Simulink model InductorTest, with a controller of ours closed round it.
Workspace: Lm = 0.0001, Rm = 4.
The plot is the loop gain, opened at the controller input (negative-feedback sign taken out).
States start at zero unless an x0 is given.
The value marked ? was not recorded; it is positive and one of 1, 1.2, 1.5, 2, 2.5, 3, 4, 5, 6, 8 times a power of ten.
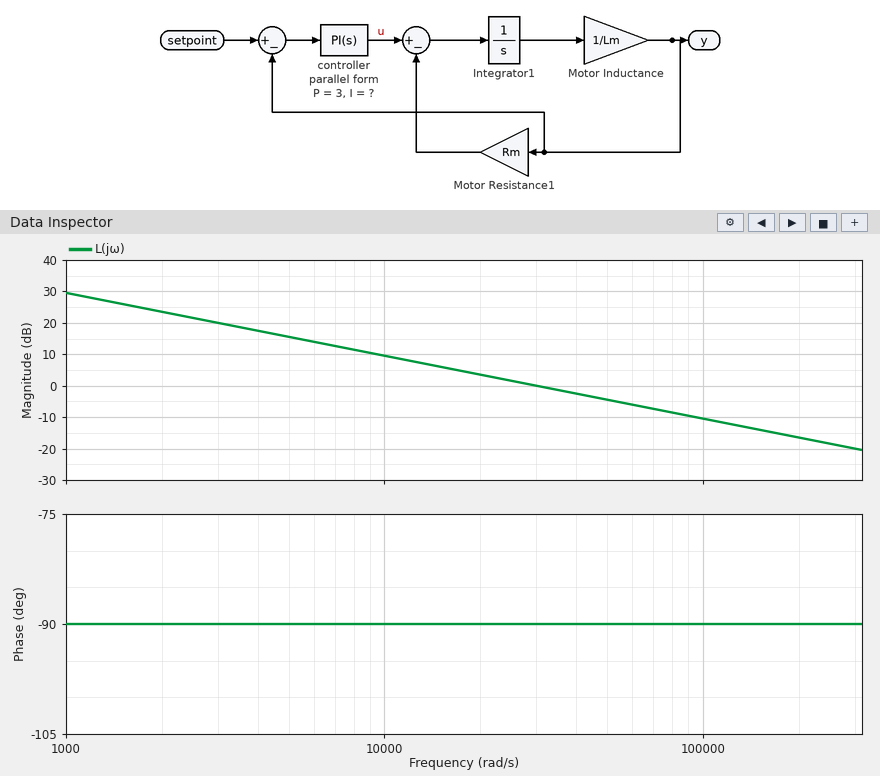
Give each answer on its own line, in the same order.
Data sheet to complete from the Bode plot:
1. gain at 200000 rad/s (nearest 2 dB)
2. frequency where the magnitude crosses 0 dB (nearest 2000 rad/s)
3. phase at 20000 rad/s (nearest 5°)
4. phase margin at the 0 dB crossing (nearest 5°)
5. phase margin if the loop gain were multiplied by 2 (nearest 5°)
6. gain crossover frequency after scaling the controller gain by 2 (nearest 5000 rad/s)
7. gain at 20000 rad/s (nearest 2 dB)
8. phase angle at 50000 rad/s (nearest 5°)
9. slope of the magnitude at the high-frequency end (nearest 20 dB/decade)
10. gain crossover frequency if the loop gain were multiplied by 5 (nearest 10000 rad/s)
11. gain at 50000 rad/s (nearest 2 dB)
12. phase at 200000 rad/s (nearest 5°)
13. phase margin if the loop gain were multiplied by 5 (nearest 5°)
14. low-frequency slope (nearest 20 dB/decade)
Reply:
-16 dB
30000 rad/s
-90°
90°
90°
60000 rad/s
4 dB
-90°
-20 dB/decade
150000 rad/s
-4 dB
-90°
90°
-20 dB/decade
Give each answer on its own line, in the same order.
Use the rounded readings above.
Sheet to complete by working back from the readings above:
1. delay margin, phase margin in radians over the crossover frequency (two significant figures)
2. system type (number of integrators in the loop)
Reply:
0.000052 s
1
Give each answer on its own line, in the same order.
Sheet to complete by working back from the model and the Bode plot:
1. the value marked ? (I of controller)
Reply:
120000
